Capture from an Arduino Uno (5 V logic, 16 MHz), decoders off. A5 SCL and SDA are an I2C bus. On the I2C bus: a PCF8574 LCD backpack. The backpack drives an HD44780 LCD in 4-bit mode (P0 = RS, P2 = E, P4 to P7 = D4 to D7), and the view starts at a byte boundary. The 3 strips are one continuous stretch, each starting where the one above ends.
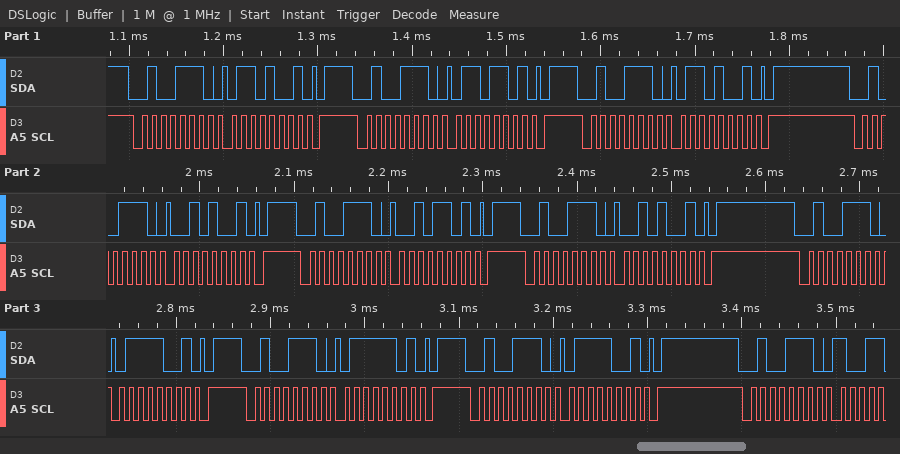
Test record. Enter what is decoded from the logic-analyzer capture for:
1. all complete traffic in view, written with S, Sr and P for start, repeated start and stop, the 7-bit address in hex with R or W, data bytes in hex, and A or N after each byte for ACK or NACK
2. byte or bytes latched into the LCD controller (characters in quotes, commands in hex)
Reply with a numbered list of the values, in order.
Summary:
1. S 27W A 69 A P S 27W A 6D A P S 27W A 69 A P S 27W A 29 A P S 27W A 2D A P S 27W A 29 A P S 27W A 79 A P S 27W A 7D A P S 27W A 79 A P S 27W A
2. 'b'
